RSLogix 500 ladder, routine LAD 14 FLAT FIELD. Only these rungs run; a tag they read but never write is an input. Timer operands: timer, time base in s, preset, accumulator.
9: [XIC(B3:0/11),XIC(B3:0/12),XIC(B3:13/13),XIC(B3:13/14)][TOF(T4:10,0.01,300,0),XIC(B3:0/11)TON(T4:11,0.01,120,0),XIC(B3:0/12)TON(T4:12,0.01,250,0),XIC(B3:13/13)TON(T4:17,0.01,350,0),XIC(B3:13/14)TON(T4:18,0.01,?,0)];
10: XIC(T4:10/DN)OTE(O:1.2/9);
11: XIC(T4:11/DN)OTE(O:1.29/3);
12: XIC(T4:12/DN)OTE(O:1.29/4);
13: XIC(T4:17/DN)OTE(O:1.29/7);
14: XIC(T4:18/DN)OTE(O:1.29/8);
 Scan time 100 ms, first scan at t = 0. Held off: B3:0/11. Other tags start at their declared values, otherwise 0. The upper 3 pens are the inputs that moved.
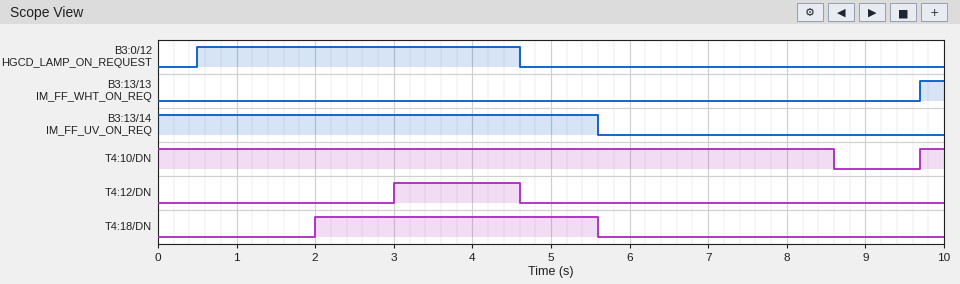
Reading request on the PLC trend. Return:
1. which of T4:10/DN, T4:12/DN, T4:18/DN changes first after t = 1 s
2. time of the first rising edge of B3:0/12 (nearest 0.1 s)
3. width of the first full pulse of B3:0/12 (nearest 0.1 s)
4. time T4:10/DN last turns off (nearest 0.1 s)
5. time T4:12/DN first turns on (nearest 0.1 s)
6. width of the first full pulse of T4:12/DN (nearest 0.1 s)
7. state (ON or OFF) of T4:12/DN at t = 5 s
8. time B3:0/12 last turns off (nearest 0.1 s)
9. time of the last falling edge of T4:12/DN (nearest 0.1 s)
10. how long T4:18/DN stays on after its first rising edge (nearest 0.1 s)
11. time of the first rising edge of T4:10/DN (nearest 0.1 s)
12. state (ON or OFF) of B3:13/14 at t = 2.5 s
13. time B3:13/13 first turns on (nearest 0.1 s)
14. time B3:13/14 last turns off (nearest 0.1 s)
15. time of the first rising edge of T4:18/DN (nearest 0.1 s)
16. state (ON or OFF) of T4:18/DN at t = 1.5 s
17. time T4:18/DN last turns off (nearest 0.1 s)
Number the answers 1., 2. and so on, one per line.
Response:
1. T4:18/DN
2. 0.5 s
3. 4.1 s
4. 8.6 s
5. 3.0 s
6. 1.6 s
7. OFF
8. 4.6 s
9. 4.6 s
10. 3.6 s
11. 9.7 s
12. ON
13. 9.7 s
14. 5.6 s
15. 2.0 s
16. OFF
17. 5.6 s
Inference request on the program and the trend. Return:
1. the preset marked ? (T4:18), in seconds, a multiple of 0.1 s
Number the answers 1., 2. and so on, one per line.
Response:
1. 2.0 s
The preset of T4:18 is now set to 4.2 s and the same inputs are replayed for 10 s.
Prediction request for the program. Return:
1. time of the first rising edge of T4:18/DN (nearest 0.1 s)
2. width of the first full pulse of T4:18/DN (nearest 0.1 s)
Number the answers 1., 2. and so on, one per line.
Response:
1. 4.2 s
2. 1.4 s
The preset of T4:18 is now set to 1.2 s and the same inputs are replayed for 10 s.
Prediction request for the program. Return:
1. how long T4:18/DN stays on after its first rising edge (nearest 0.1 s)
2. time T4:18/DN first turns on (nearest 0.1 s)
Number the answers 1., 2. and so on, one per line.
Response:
1. 4.4 s
2. 1.2 s
